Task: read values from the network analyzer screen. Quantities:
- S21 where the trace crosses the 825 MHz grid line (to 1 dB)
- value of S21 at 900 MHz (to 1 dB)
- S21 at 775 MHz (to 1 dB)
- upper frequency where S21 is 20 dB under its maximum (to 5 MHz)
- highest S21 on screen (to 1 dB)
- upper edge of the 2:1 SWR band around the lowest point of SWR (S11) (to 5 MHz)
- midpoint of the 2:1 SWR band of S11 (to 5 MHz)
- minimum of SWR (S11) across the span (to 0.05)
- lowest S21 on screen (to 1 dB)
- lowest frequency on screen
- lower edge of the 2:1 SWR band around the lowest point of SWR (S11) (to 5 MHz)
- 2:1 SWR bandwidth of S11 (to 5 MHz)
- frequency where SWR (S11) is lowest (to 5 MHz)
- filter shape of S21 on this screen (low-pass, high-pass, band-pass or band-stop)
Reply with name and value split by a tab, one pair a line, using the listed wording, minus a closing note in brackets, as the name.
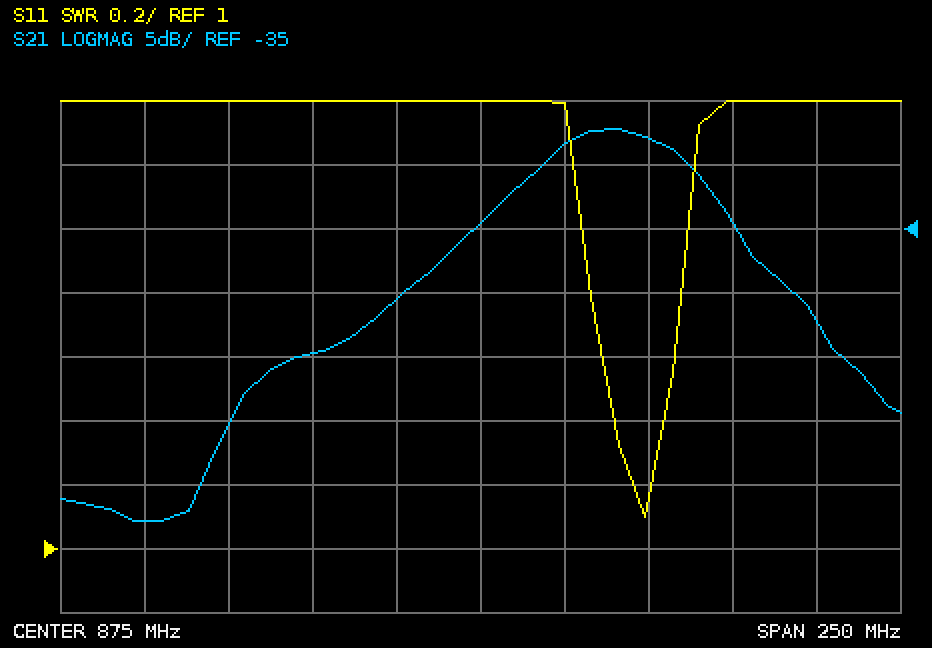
S21 where the trace crosses the 825 MHz grid line	-45 dB
value of S21 at 900 MHz	-28 dB
S21 at 775 MHz	-58 dB
upper frequency where S21 is 20 dB under its maximum	990 MHz
highest S21 on screen	-27 dB
upper edge of the 2:1 SWR band around the lowest point of SWR (S11)	935 MHz
midpoint of the 2:1 SWR band of S11	920 MHz
minimum of SWR (S11) across the span	1.10
lowest S21 on screen	-58 dB
lowest frequency on screen	750 MHz
lower edge of the 2:1 SWR band around the lowest point of SWR (S11)	905 MHz
2:1 SWR bandwidth of S11	30 MHz
frequency where SWR (S11) is lowest	925 MHz
filter shape of S21 on this screen	band-pass
